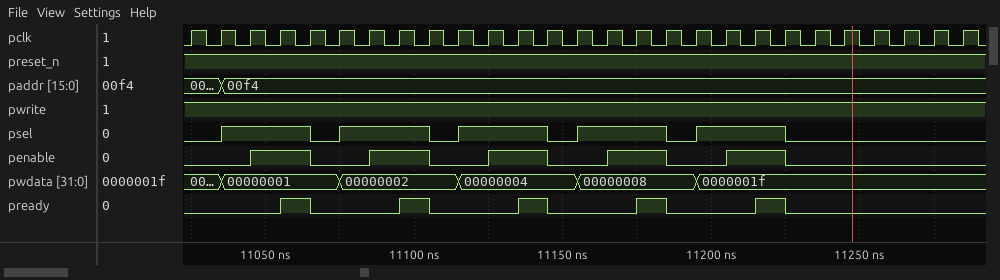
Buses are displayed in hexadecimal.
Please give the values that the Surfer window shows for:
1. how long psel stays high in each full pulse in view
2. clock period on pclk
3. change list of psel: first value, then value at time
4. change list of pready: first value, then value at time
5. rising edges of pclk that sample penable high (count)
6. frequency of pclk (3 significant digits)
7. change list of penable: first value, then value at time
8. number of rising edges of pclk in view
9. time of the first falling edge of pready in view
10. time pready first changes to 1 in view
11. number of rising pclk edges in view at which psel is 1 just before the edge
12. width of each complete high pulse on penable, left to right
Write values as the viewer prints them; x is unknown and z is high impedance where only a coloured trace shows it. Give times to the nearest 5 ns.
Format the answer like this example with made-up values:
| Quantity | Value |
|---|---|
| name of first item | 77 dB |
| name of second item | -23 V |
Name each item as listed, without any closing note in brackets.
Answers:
| Quantity | Value |
|---|---|
| how long psel stays high in each full pulse in view | 30 ns, 30 ns, 30 ns, 30 ns, 30 ns |
| clock period on pclk | 10 ns |
| change list of psel: first value, then value at time | 0, 1 at 11035 ns, 0 at 11065 ns, 1 at 11075 ns, 0 at 11105 ns, 1 at 11115 ns, 0 at 11145 ns, 1 at 11155 ns, 0 at 11185 ns, 1 at 11195 ns, 0 at 11225 ns |
| change list of pready: first value, then value at time | 0, 1 at 11055 ns, 0 at 11065 ns, 1 at 11095 ns, 0 at 11105 ns, 1 at 11135 ns, 0 at 11145 ns, 1 at 11175 ns, 0 at 11185 ns, 1 at 11215 ns, 0 at 11225 ns |
| rising edges of pclk that sample penable high | 10 |
| frequency of pclk | 100 MHz |
| change list of penable: first value, then value at time | 0, 1 at 11045 ns, 0 at 11065 ns, 1 at 11085 ns, 0 at 11105 ns, 1 at 11125 ns, 0 at 11145 ns, 1 at 11165 ns, 0 at 11185 ns, 1 at 11205 ns, 0 at 11225 ns |
| number of rising edges of pclk in view | 27 |
| time of the first falling edge of pready in view | 11065 ns |
| time pready first changes to 1 in view | 11055 ns |
| number of rising pclk edges in view at which psel is 1 just before the edge | 15 |
| width of each complete high pulse on penable, left to right | 20 ns, 20 ns, 20 ns, 20 ns, 20 ns |
